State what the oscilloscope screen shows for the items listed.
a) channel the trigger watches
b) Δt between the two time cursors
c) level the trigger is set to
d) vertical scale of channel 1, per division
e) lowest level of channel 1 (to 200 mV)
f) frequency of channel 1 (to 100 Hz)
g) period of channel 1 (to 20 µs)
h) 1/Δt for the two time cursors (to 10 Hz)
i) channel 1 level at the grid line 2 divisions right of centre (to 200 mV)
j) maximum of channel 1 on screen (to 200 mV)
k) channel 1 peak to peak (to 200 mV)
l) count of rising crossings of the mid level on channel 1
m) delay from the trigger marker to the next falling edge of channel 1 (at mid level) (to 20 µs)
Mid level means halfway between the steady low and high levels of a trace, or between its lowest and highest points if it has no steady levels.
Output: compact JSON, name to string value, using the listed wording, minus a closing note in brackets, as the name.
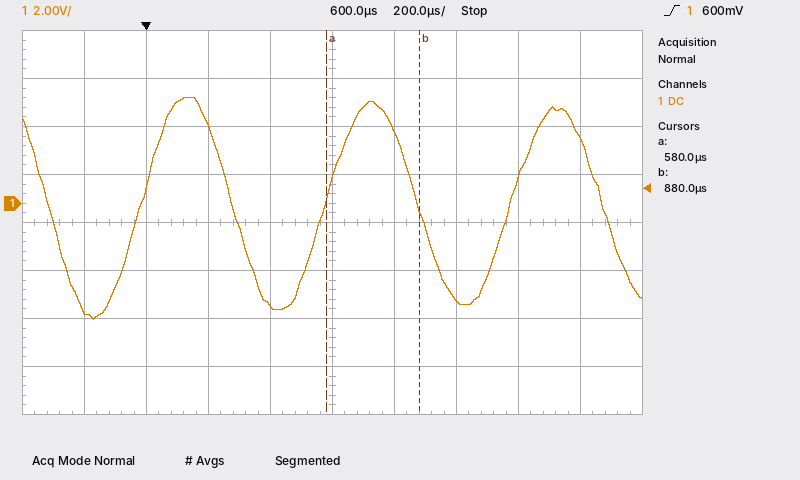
{"channel the trigger watches": "channel 1", "Δt between the two time cursors": "300 µs", "level the trigger is set to": "600 mV", "vertical scale of channel 1, per division": "2 V", "lowest level of channel 1": "-4.8 V", "frequency of channel 1": "1.7 kHz", "period of channel 1": "600 µs", "1/Δt for the two time cursors": "3.33 kHz", "channel 1 level at the grid line 2 divisions right of centre": "-4.0 V", "maximum of channel 1 on screen": "4.4 V", "channel 1 peak to peak": "9.2 V", "count of rising crossings of the mid level on channel 1": "3", "delay from the trigger marker to the next falling edge of channel 1 (at mid level)": "280 µs"}
